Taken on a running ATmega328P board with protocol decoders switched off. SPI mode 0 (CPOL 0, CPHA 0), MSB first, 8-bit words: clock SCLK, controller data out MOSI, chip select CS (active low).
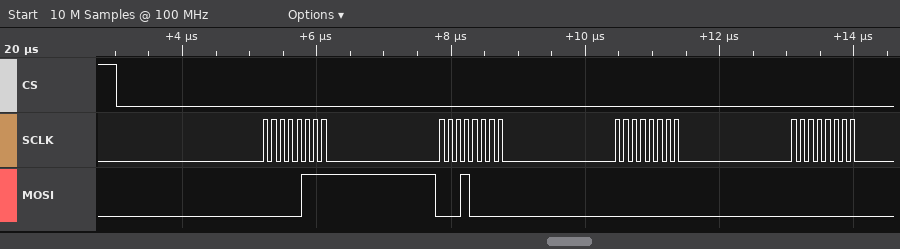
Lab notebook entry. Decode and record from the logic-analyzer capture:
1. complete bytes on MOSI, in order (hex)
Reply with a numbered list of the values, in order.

1. 07 10 00 00
